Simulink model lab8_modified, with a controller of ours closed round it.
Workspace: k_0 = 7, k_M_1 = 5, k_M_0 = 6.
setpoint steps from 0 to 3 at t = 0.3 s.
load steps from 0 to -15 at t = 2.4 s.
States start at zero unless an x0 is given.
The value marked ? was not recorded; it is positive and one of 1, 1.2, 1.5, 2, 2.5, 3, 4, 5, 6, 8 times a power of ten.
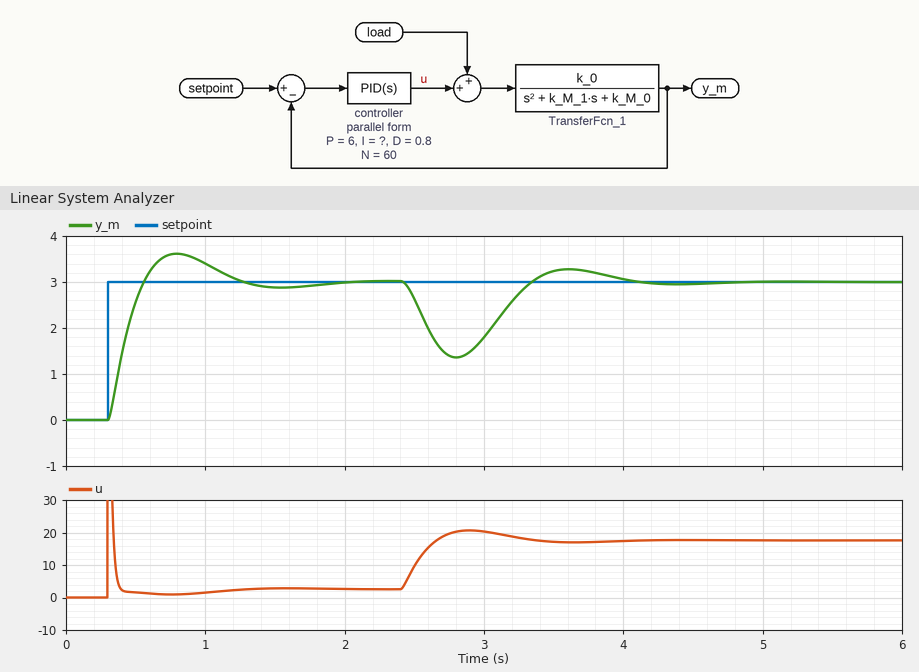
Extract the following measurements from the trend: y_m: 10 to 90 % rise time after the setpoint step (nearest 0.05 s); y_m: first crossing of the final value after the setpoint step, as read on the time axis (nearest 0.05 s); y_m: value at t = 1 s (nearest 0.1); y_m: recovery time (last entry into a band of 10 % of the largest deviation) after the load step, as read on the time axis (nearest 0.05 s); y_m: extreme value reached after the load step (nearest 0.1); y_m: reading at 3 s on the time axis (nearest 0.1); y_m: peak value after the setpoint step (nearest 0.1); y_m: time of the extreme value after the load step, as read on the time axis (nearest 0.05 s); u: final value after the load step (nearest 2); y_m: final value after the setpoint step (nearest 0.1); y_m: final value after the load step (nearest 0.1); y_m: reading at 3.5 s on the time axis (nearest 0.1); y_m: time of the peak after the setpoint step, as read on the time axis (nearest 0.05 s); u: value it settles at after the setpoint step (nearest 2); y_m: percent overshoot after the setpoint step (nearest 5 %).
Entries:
0.20 s
0.55 s
3.4
3.85 s
1.4
1.8
3.6
2.80 s
18
3.0
3.0
3.2
0.80 s
2
20 %
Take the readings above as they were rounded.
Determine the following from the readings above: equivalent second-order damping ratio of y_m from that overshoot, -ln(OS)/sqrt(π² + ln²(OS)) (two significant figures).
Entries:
0.46
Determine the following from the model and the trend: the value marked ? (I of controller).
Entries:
20
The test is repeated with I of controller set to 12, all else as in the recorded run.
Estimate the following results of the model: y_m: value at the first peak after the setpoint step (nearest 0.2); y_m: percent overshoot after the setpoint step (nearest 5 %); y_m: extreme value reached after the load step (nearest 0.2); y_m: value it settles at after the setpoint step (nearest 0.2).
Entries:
3.4
10 %
1.2
3.0
